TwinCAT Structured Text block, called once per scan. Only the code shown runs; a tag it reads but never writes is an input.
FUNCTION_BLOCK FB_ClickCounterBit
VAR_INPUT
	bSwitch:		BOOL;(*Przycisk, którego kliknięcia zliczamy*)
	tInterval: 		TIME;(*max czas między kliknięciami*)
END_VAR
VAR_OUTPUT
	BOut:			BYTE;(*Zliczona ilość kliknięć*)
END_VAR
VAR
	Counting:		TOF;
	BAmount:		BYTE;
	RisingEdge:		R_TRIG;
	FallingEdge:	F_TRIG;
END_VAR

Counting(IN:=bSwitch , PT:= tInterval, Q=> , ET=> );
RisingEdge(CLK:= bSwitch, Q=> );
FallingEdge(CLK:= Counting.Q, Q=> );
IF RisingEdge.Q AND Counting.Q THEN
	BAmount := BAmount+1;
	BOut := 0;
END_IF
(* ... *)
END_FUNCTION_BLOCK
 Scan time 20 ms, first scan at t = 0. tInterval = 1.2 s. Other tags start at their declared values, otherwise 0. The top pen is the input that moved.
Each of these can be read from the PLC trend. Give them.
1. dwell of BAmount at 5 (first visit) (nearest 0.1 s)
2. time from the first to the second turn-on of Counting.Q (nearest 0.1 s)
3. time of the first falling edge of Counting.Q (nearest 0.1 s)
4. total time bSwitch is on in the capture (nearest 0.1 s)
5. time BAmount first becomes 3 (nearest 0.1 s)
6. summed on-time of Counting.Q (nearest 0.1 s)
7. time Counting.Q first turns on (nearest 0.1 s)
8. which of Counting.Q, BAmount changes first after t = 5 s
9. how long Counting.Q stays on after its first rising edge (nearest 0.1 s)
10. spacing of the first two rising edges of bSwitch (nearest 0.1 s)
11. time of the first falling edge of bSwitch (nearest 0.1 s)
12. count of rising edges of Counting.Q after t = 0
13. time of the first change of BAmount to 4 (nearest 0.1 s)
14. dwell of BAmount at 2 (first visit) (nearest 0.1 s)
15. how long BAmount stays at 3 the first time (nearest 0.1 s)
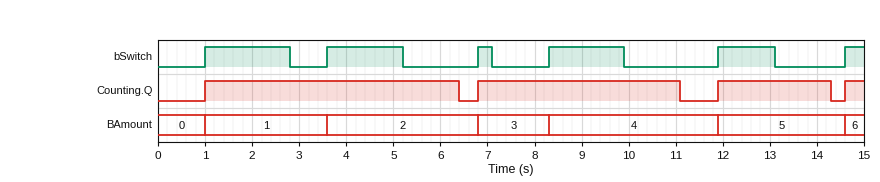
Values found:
2.7 s
5.8 s
6.4 s
6.9 s
6.8 s
12.5 s
1.0 s
Counting.Q
5.4 s
2.6 s
2.8 s
4
8.3 s
3.2 s
1.5 s
